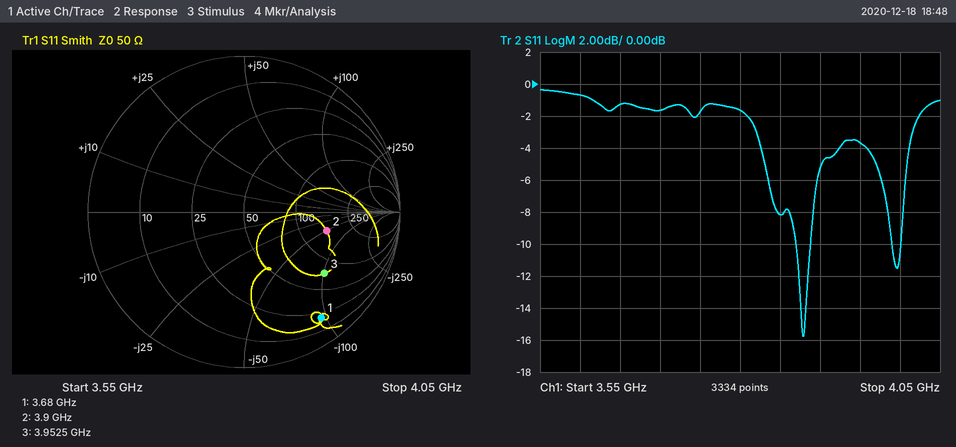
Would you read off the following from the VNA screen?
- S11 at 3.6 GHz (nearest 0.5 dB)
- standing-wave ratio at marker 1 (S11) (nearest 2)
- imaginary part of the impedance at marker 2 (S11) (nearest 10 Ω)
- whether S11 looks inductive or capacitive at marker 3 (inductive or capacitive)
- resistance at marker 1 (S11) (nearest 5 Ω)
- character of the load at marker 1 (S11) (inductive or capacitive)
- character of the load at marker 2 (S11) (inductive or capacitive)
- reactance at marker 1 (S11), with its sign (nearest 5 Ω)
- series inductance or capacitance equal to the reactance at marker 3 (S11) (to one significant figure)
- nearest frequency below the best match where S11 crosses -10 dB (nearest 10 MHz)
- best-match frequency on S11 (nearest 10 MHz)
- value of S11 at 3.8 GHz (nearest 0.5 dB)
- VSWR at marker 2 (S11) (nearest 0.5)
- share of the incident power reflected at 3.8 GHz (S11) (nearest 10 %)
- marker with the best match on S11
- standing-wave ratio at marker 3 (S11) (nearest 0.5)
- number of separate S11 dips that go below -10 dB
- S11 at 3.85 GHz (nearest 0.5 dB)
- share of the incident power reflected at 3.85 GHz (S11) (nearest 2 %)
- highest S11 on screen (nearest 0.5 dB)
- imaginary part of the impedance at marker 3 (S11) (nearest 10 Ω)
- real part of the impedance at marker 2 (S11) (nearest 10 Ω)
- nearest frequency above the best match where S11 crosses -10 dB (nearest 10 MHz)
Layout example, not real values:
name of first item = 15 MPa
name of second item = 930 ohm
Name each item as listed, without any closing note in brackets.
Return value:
S11 at 3.6 GHz = -0.5 dB
standing-wave ratio at marker 1 (S11) = 12
imaginary part of the impedance at marker 2 (S11) = -50 Ω
whether S11 looks inductive or capacitive at marker 3 = capacitive
resistance at marker 1 (S11) = 20 Ω
character of the load at marker 1 (S11) = capacitive
character of the load at marker 2 (S11) = capacitive
reactance at marker 1 (S11), with its sign = -95 Ω
series inductance or capacitance equal to the reactance at marker 3 (S11) = 400 fF
nearest frequency below the best match where S11 crosses -10 dB = 3.87 GHz
best-match frequency on S11 = 3.88 GHz
value of S11 at 3.8 GHz = -1.5 dB
VSWR at marker 2 (S11) = 3.5
share of the incident power reflected at 3.8 GHz (S11) = 70 %
marker with the best match on S11 = marker 2
standing-wave ratio at marker 3 (S11) = 4.5
number of separate S11 dips that go below -10 dB = 2
S11 at 3.85 GHz = -8.0 dB
share of the incident power reflected at 3.85 GHz (S11) = 16 %
highest S11 on screen = -0.5 dB
imaginary part of the impedance at marker 3 (S11) = -100 Ω
real part of the impedance at marker 2 (S11) = 150 Ω
nearest frequency above the best match where S11 crosses -10 dB = 3.89 GHz
